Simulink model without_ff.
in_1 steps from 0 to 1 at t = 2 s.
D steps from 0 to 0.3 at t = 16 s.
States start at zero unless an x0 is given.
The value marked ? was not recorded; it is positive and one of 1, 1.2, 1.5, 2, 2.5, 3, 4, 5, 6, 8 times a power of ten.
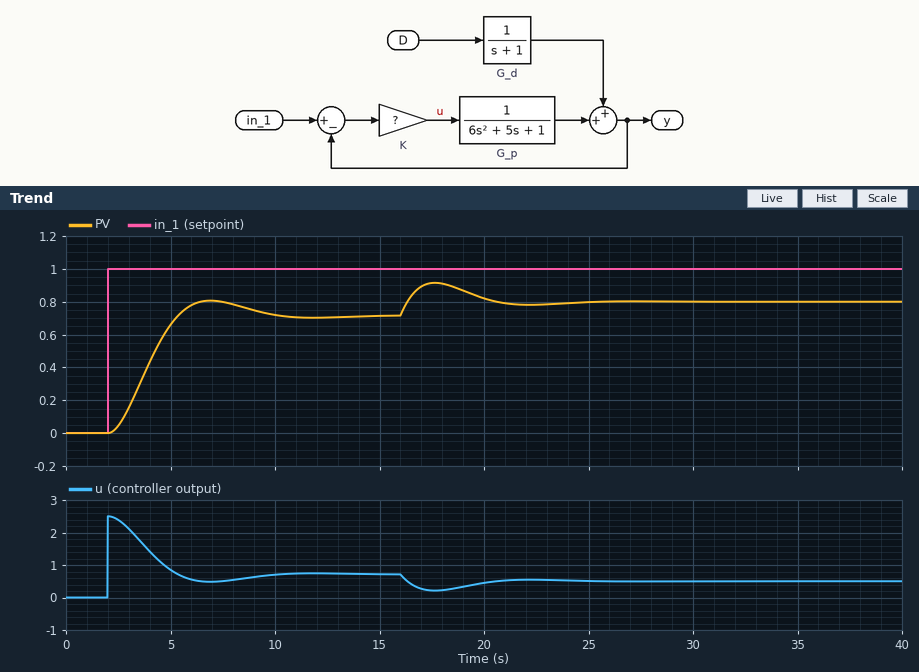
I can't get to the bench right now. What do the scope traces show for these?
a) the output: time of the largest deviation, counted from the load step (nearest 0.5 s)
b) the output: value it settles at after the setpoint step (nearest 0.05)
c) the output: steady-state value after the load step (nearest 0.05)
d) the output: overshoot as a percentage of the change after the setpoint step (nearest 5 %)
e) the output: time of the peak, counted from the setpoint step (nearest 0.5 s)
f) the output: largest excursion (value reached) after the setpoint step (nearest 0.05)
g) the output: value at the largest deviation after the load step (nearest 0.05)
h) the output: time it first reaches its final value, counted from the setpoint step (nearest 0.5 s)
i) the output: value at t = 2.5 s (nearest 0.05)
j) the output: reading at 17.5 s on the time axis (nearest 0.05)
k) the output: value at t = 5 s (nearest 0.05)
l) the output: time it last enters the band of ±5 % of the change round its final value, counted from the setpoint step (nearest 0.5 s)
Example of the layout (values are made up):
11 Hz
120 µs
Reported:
1.5 s
0.70
0.80
15 %
5.0 s
0.80
0.90
3.5 s
0.05
0.90
0.65
7.0 s
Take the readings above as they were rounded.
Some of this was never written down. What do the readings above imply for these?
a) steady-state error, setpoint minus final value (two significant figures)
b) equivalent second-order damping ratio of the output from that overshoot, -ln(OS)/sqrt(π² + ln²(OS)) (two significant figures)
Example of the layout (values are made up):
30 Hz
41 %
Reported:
0.30
0.52
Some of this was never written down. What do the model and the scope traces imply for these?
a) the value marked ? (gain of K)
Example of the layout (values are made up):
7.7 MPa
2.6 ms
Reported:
2.5
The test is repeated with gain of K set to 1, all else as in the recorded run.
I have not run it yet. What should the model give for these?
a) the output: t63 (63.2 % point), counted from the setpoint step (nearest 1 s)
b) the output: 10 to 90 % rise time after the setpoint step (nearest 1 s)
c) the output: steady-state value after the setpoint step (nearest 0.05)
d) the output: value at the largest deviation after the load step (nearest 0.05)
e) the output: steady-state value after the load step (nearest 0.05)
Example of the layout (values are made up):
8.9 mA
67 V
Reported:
3 s
4 s
0.50
0.75
0.65
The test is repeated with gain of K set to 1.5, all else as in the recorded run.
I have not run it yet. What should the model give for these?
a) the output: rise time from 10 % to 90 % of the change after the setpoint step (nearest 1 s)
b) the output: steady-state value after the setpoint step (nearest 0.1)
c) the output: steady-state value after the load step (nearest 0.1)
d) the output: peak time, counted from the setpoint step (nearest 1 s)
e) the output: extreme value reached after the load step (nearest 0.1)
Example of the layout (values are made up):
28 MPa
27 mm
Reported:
3 s
0.6
0.7
6 s
0.8
